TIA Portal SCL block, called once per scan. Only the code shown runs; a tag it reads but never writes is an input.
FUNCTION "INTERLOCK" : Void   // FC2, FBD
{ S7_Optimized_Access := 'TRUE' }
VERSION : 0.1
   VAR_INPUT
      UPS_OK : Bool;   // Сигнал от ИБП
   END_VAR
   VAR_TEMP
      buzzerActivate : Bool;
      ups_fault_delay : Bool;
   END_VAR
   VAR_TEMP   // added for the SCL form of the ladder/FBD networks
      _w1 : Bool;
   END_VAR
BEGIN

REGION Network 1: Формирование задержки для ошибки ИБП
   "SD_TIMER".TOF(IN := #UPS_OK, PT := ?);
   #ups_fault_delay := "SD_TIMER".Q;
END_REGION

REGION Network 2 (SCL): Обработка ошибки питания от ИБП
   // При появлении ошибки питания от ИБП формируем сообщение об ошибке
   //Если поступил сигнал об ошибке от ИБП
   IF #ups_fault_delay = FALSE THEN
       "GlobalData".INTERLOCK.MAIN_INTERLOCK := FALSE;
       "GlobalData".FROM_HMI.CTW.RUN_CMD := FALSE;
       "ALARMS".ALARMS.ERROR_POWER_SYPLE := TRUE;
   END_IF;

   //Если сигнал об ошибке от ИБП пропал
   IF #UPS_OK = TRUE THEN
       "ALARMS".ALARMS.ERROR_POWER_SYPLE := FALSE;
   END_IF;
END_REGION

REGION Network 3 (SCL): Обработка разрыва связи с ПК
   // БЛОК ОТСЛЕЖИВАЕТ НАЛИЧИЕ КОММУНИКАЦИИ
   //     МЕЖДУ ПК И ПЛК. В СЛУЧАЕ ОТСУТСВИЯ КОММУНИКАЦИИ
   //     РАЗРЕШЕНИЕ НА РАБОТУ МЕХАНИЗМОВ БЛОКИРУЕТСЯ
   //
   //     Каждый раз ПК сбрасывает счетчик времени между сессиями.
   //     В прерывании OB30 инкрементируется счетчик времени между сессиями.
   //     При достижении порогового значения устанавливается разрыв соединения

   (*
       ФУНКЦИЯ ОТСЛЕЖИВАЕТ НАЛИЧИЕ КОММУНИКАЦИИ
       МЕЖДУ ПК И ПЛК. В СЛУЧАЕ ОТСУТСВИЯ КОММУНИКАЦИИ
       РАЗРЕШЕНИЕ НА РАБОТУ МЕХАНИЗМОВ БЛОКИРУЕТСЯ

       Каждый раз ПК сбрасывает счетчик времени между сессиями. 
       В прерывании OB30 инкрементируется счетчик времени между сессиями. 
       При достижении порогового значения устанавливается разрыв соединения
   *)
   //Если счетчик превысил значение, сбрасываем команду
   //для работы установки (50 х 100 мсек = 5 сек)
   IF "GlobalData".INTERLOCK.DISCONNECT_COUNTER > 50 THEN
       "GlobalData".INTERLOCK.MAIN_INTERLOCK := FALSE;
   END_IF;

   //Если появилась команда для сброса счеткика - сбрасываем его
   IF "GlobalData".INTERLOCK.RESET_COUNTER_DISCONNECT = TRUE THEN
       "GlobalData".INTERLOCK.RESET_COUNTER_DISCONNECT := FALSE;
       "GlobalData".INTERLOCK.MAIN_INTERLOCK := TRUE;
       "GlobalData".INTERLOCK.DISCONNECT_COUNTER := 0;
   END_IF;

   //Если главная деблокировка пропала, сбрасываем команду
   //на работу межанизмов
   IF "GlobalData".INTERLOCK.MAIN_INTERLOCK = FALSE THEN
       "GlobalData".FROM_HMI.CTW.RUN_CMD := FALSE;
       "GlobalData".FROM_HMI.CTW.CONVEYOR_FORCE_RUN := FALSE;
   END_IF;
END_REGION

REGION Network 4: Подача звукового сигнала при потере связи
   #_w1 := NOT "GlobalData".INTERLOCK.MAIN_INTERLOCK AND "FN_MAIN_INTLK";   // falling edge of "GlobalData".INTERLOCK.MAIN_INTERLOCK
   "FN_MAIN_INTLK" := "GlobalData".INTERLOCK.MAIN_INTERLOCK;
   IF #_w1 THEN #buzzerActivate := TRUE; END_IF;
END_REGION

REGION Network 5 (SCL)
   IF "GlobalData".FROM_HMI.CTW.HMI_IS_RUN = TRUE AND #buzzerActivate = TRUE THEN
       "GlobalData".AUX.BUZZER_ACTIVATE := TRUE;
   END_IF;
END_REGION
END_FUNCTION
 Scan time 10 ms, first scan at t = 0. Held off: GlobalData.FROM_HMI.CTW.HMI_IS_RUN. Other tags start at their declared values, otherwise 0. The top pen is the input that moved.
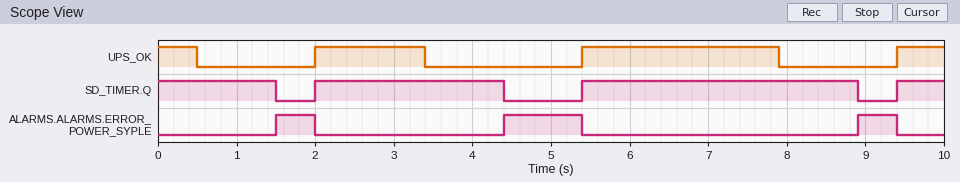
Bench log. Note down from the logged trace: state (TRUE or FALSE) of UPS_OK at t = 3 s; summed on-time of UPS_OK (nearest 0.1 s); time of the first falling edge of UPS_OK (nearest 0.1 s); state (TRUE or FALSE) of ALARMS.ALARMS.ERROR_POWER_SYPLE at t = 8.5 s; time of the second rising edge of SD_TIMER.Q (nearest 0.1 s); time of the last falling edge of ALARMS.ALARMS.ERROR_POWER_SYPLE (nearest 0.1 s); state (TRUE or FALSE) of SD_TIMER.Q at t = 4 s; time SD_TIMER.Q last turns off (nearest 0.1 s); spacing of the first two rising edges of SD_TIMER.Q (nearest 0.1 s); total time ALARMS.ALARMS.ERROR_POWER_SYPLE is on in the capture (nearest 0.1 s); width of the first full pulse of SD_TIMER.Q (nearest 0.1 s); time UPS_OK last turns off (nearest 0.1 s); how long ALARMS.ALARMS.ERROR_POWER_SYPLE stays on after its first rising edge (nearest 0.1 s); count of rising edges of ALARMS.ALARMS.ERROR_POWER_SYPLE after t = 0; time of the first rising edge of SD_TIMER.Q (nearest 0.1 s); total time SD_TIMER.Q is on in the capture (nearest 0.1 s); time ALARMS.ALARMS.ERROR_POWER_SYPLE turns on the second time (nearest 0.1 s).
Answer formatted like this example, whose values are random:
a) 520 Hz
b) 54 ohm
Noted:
a) TRUE
b) 5.0 s
c) 0.5 s
d) FALSE
e) 5.4 s
f) 9.4 s
g) TRUE
h) 8.9 s
i) 3.4 s
j) 2.0 s
k) 2.4 s
l) 7.9 s
m) 0.5 s
n) 3
o) 2.0 s
p) 8.0 s
q) 4.4 s
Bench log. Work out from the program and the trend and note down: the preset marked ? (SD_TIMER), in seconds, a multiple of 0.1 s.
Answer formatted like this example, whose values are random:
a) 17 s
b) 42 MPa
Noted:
a) 1.0 s
